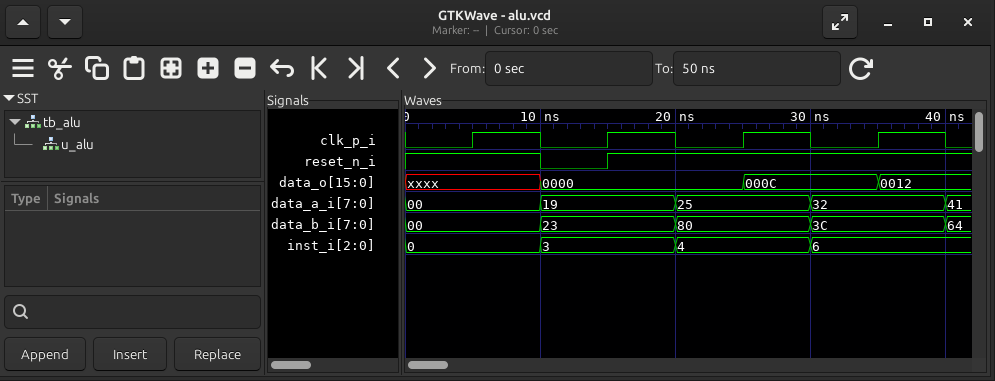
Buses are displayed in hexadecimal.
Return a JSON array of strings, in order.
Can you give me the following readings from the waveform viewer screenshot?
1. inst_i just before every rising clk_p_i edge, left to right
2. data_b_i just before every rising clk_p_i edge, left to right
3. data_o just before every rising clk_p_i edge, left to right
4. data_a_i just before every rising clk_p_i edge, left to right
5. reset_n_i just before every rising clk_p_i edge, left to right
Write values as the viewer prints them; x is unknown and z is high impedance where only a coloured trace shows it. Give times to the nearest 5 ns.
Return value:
["0, 3, 4, 6", "00, 23, 80, 3C", "xxxx, 0000, 0000, 000C", "00, 19, 25, 32", "1 0 1 1"]
